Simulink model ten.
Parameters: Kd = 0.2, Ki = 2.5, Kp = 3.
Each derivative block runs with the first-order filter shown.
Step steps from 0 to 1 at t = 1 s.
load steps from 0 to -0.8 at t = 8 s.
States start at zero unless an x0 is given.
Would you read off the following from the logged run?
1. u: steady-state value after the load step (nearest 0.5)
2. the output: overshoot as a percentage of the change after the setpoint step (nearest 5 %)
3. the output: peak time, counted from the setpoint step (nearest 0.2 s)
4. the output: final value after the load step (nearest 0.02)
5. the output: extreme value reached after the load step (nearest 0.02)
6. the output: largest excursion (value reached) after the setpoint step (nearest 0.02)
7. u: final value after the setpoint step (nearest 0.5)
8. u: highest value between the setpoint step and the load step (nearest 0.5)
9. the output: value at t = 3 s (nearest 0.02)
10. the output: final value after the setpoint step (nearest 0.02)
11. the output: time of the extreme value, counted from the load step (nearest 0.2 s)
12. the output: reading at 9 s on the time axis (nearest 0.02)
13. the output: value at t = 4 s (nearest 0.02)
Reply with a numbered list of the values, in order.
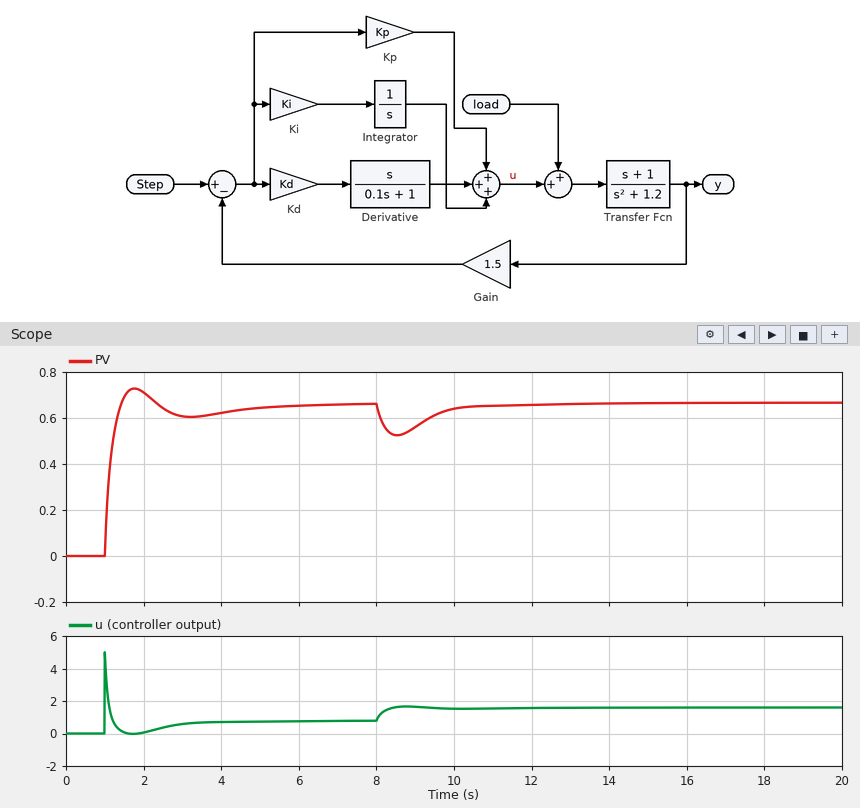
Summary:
1. 1.5
2. 10 %
3. 0.8 s
4. 0.66
5. 0.52
6. 0.72
7. 1.0
8. 5.0
9. 0.60
10. 0.66
11. 0.6 s
12. 0.56
13. 0.62
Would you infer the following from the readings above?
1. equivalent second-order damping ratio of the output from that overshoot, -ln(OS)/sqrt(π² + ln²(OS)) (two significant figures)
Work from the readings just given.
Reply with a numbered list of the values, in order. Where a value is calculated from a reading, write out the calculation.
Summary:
1. ln(0.1) = -2.303; 2.303 / sqrt(9.870 + 5.302) = 0.59
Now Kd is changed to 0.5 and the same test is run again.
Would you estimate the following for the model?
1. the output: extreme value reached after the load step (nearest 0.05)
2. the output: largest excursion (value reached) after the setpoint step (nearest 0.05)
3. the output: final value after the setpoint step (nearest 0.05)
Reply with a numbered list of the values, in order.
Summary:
1. 0.55
2. 0.70
3. 0.65
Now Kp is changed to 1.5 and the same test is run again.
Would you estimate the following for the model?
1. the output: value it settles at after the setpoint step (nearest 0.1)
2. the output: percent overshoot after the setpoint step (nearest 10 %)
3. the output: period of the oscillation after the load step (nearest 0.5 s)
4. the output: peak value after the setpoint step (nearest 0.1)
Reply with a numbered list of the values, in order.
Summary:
1. 0.7
2. 20 %
3. 3.0 s
4. 0.8
